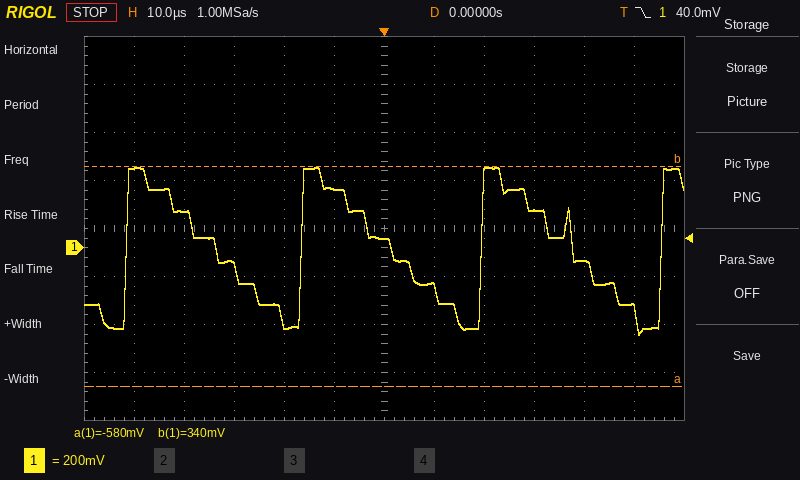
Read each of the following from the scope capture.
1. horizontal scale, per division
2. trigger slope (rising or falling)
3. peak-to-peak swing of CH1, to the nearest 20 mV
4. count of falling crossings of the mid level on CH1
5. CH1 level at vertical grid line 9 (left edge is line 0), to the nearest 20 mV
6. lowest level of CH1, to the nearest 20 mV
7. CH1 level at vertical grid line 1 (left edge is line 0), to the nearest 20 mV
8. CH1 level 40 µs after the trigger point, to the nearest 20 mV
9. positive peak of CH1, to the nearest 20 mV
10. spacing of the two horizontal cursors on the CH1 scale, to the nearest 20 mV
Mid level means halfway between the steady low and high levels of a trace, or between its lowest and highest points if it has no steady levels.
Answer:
10 µs
falling
700 mV
3
160 mV
-360 mV
340 mV
-60 mV
340 mV
920 mV
